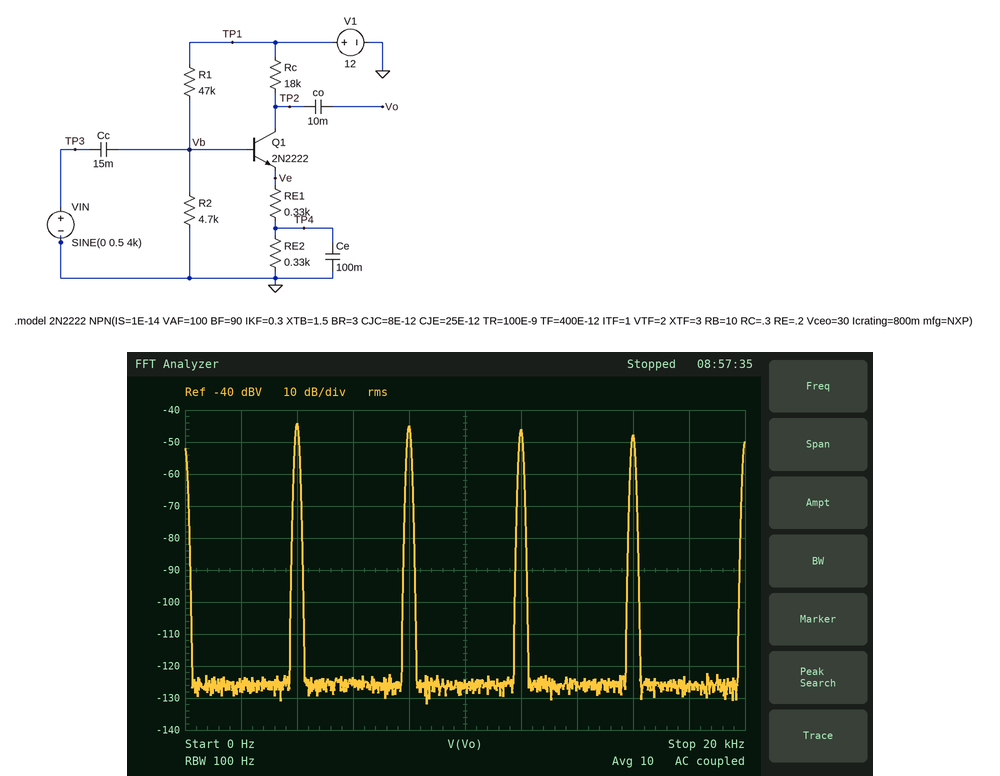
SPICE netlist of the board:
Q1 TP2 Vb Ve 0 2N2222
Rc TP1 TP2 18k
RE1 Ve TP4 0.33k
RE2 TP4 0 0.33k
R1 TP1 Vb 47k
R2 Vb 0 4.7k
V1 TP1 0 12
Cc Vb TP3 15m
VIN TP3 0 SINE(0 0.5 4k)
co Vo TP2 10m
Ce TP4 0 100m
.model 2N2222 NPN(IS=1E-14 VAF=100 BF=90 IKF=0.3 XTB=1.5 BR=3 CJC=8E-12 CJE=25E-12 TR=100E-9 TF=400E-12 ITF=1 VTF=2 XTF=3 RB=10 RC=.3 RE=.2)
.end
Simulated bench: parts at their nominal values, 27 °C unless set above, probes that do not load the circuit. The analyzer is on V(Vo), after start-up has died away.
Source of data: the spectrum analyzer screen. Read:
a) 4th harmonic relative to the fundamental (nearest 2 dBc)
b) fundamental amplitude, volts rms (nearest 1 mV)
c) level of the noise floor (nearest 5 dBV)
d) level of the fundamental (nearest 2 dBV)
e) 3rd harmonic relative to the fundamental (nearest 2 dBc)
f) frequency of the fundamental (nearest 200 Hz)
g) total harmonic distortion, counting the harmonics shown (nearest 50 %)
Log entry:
-4 dBc
6 mV
-125 dBV
-44 dBV
-2 dBc
4.0 kHz
150 %
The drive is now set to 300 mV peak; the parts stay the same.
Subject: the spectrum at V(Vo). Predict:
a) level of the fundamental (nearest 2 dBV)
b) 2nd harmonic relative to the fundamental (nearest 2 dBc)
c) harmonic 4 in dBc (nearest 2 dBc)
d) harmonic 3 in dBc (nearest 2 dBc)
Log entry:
-70 dBV
-40 dBc
-44 dBc
-42 dBc
